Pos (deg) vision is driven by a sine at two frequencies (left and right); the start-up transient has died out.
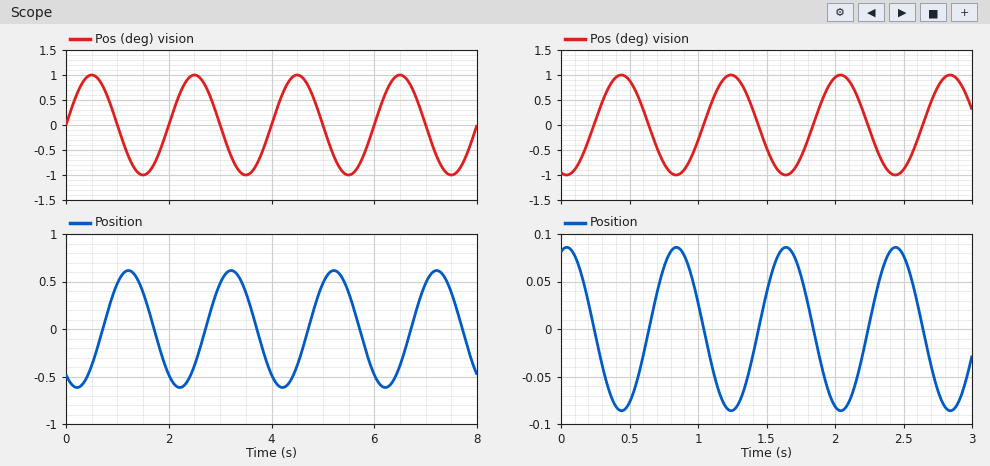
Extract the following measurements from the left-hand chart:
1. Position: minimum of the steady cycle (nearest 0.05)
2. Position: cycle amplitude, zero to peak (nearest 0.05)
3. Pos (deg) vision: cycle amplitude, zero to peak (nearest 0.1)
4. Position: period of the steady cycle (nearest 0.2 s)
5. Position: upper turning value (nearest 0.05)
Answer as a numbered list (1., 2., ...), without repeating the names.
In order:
1. -0.60
2. 0.60
3. 1.0
4. 2.0 s
5. 0.60
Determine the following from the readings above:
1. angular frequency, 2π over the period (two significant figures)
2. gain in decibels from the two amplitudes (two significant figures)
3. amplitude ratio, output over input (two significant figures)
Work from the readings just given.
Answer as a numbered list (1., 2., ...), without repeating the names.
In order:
1. 3.1 rad/s
2. -4.4 dB
3. 0.60
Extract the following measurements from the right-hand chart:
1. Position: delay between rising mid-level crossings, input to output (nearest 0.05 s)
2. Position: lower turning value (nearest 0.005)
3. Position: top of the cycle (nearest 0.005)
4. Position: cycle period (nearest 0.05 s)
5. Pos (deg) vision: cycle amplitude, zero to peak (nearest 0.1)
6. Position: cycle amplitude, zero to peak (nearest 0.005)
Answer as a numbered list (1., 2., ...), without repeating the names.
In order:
1. 0.40 s
2. -0.085
3. 0.085
4. 0.80 s
5. 1.0
6. 0.085
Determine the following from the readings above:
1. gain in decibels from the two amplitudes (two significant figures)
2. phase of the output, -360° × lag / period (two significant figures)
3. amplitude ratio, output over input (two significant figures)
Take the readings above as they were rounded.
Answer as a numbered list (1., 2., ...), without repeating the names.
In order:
1. -21 dB
2. -180°
3. 0.085
